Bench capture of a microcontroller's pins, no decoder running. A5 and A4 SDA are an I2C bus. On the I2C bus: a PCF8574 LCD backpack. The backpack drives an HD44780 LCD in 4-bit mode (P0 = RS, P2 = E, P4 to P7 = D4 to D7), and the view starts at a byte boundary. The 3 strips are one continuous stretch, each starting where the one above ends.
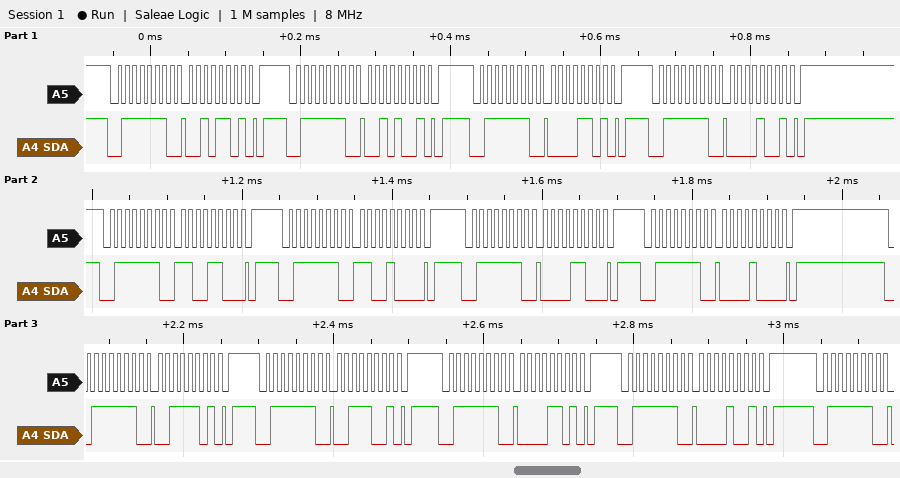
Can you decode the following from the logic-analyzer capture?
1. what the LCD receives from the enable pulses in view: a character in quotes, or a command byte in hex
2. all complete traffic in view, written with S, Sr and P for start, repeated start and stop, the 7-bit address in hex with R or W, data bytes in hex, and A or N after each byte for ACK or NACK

' ' 0xC0 '0'
S 3FW A 2D A P S 3FW A 29 A P S 3FW A 0D A P S 3FW A 09 A P S 3FW A CC A P S 3FW A C8 A P S 3FW A 0C A P S 3FW A 08 A P S 3FW A 3D A P S 3FW A 39 A P S 3FW A 0D A P S 3FW A 09 A P S 3FW A
